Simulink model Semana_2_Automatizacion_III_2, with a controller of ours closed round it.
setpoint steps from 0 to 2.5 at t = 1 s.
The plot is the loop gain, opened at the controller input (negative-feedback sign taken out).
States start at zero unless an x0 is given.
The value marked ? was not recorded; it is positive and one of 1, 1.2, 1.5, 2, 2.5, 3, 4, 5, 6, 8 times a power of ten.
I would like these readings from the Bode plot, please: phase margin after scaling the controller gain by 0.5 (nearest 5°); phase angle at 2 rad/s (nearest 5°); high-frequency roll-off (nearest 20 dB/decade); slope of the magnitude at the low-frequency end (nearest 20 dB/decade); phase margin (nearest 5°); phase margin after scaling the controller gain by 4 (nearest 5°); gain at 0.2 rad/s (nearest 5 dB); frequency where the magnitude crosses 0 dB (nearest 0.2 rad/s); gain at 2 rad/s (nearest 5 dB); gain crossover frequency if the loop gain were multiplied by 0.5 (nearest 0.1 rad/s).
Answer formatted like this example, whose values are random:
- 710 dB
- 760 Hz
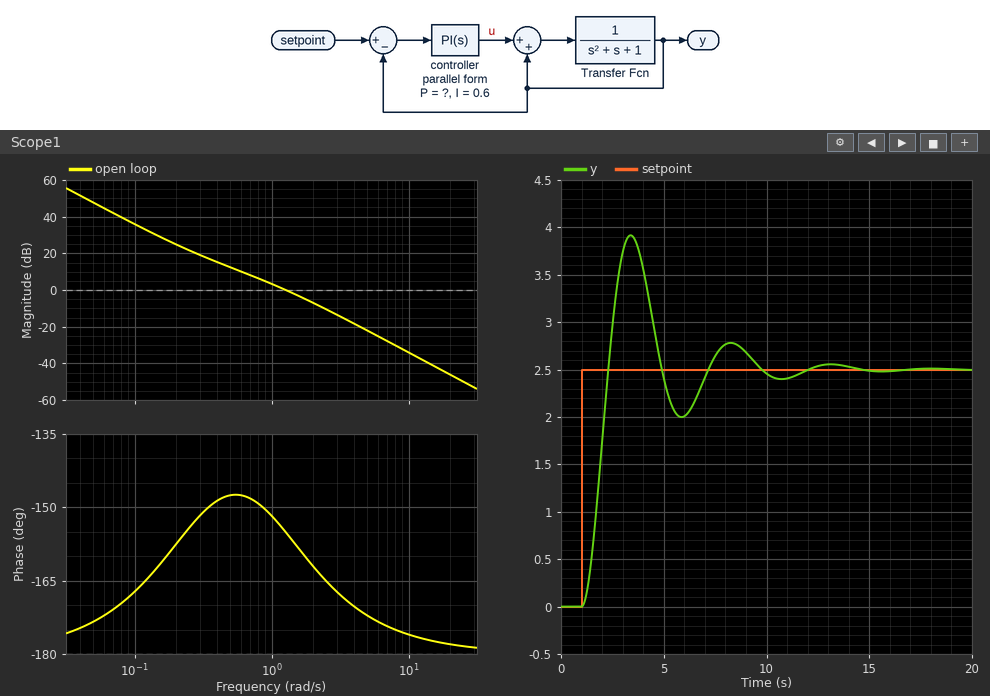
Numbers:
- 30°
- -160°
- -40 dB/decade
- -40 dB/decade
- 25°
- 15°
- 25 dB
- 1.2 rad/s
- -5 dB
- 0.8 rad/s
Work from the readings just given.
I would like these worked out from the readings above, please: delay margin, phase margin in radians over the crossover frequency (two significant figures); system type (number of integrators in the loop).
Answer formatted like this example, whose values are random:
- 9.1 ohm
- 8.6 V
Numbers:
- 0.36 s
- 2
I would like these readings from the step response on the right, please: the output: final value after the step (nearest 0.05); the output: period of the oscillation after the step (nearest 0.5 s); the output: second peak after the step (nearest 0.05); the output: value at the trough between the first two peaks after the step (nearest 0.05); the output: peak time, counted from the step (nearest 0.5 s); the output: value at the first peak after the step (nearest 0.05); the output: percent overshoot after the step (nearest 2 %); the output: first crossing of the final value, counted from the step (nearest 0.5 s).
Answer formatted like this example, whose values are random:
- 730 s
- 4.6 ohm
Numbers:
- 2.50
- 5.0 s
- 2.80
- 2.00
- 2.5 s
- 3.90
- 56 %
- 1.5 s
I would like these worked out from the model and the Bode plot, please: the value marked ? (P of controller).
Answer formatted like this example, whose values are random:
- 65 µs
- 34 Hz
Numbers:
- 2
